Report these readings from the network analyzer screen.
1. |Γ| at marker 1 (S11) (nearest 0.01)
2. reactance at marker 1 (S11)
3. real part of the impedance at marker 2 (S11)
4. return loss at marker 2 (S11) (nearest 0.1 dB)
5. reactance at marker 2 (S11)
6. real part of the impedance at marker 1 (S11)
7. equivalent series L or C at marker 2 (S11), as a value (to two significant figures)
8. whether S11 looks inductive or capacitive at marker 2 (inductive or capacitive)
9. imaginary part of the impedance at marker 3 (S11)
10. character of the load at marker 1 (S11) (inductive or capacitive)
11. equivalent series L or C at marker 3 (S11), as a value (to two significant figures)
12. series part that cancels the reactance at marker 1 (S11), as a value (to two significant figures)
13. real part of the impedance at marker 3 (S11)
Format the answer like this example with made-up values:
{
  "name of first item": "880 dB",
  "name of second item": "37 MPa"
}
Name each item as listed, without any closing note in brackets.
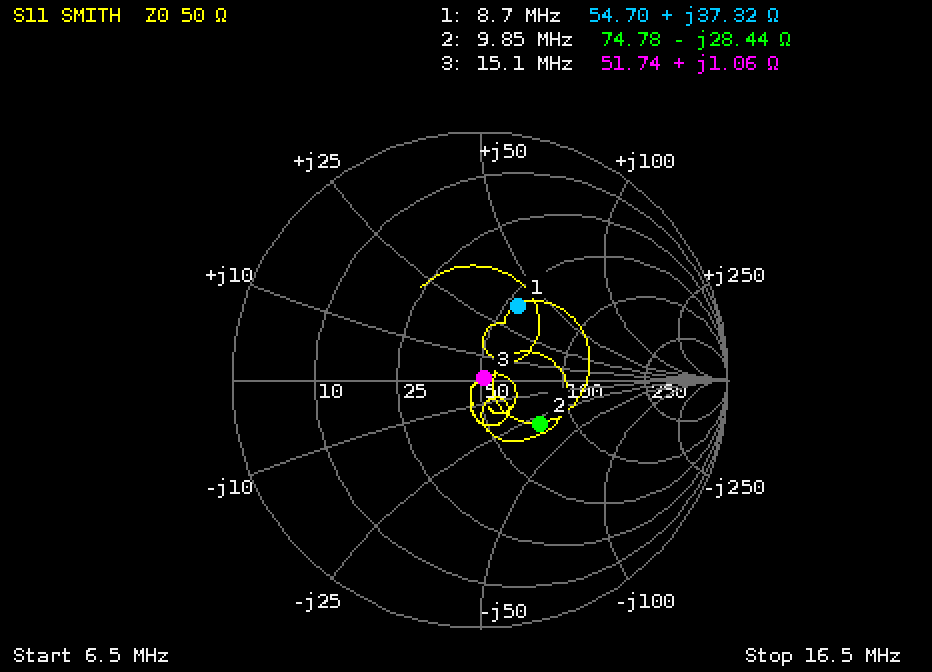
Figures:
{
  "|Γ| at marker 1 (S11)": "0.34",
  "reactance at marker 1": "+37.32 Ω",
  "real part of the impedance at marker 2": "74.78 Ω",
  "return loss at marker 2 (S11)": "10.6 dB",
  "reactance at marker 2": "-28.44 Ω",
  "real part of the impedance at marker 1": "54.70 Ω",
  "equivalent series L or C at marker 2 (S11), as a value": "570 pF",
  "whether S11 looks inductive or capacitive at marker 2": "capacitive",
  "imaginary part of the impedance at marker 3": "+1.06 Ω",
  "character of the load at marker 1 (S11)": "inductive",
  "equivalent series L or C at marker 3 (S11), as a value": "11 nH",
  "series part that cancels the reactance at marker 1 (S11), as a value": "490 pF",
  "real part of the impedance at marker 3": "51.74 Ω"
}
